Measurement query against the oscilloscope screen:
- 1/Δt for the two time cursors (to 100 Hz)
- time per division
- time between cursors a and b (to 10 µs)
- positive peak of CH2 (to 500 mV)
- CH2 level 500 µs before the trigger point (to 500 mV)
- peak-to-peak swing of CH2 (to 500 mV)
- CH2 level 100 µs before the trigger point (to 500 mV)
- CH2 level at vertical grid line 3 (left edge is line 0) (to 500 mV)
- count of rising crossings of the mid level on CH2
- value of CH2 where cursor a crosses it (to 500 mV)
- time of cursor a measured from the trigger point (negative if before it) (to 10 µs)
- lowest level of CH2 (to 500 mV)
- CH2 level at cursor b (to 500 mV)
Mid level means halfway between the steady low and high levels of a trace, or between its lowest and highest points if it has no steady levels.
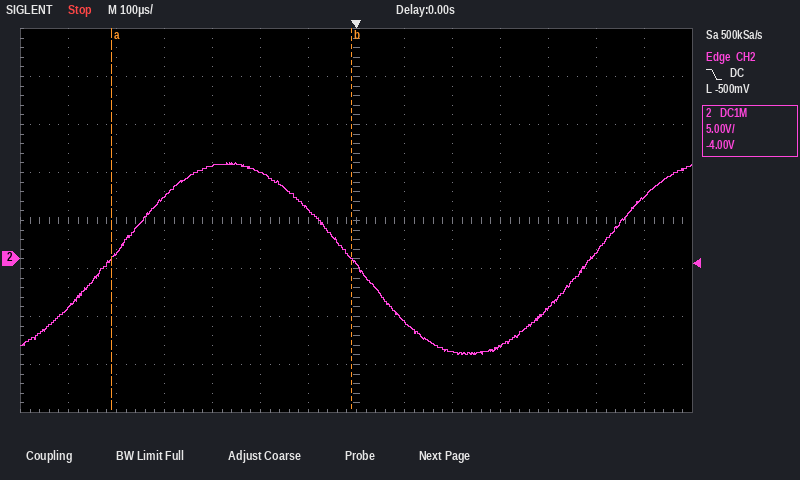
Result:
2.0 kHz
100 µs
500 µs
10.0 V
500 mV
20.0 V
5.0 V
6.5 V
2
0.0 V
-510 µs
-10.0 V
0.0 V
